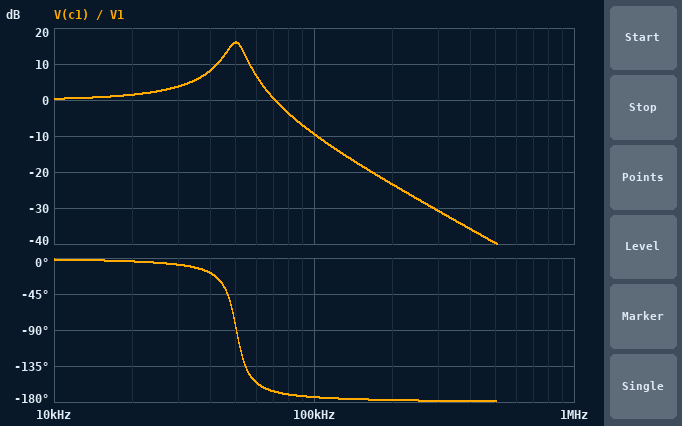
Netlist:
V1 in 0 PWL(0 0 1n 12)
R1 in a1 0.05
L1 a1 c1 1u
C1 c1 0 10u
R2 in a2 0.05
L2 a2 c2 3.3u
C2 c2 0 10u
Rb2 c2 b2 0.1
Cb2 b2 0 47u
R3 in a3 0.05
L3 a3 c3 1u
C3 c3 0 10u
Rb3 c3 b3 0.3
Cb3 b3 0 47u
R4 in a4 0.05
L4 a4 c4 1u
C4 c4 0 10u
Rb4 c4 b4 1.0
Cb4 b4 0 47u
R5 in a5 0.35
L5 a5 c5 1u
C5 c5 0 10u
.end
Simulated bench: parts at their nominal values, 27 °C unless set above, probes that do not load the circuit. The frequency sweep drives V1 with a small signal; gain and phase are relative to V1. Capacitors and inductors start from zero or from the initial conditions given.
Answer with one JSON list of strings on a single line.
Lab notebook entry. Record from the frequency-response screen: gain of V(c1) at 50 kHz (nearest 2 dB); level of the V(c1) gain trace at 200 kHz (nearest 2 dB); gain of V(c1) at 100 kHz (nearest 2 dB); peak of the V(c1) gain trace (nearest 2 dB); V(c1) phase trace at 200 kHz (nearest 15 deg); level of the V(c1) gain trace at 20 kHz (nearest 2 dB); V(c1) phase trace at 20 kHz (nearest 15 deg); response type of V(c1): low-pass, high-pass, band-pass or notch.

["16 dB", "-24 dB", "-10 dB", "16 dB", "-180 deg", "2 dB", "0 deg", "low-pass"]
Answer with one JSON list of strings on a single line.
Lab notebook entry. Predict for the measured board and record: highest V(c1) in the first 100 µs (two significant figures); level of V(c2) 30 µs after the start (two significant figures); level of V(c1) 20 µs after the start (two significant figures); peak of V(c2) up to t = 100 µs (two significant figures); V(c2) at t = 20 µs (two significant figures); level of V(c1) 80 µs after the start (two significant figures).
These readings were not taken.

["21 V", "16 V", "4.7 V", "18 V", "11 V", "10 V"]
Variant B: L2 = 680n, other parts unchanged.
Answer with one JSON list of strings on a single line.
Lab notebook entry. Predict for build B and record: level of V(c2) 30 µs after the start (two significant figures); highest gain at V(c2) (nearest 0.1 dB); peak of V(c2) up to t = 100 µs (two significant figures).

["12 V", "1.7 dB", "14 V"]
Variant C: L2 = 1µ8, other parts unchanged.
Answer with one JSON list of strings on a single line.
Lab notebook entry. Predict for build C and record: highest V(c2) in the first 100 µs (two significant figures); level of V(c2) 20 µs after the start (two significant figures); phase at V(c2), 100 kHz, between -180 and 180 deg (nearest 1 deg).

["16 V", "14 V", "-131 deg"]
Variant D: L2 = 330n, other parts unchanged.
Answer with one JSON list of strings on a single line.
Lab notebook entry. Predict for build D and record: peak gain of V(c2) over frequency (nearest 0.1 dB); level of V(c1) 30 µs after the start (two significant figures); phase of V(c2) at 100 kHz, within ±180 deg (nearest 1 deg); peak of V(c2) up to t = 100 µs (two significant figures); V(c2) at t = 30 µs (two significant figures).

["0.2 dB", "18 V", "-102 deg", "13 V", "12 V"]
